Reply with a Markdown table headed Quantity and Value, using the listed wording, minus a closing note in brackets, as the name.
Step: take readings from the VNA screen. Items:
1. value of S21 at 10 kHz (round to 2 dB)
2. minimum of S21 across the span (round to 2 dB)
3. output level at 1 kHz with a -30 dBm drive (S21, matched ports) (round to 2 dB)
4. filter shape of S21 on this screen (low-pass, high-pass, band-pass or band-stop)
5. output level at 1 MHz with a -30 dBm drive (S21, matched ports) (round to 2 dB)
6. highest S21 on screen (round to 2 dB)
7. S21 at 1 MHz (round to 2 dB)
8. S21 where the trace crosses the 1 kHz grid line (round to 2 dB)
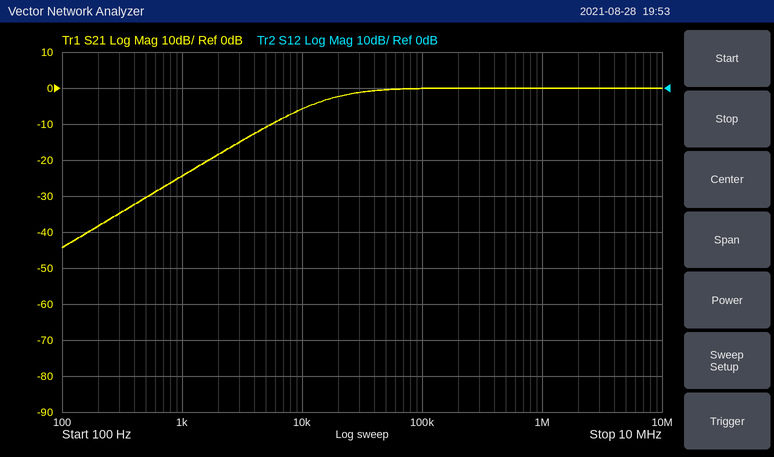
| Quantity | Value |
|---|---|
| value of S21 at 10 kHz | -6 dB |
| minimum of S21 across the span | -44 dB |
| output level at 1 kHz with a -30 dBm drive (S21, matched ports) | -54 dBm |
| filter shape of S21 on this screen | high-pass |
| output level at 1 MHz with a -30 dBm drive (S21, matched ports) | -30 dBm |
| highest S21 on screen | 0 dB |
| S21 at 1 MHz | 0 dB |
| S21 where the trace crosses the 1 kHz grid line | -24 dB |
